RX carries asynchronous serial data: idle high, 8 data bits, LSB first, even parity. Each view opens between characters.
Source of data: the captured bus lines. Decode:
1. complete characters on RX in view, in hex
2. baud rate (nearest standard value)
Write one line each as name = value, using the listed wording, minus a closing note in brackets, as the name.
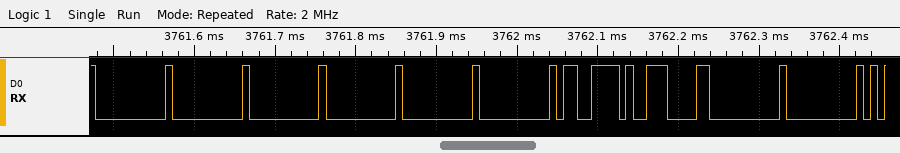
complete characters on RX in view, in hex = 00, 00, 00, 00, 00, 00, F3, 0E, 00, 00
baud rate = 115200 baud
